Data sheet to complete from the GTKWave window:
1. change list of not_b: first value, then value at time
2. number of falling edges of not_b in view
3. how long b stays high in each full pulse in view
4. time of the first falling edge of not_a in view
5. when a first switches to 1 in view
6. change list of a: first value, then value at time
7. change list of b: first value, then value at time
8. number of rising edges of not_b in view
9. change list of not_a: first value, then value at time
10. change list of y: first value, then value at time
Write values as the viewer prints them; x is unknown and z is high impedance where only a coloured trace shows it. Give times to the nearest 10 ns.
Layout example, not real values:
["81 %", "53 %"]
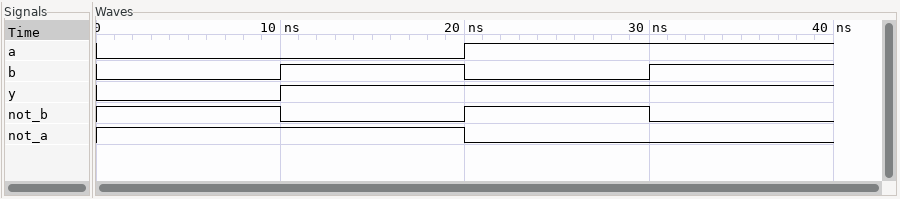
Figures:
["1, 0 at 10 ns, 1 at 20 ns, 0 at 30 ns", "2", "10 ns", "20 ns", "20 ns", "0, 1 at 20 ns", "0, 1 at 10 ns, 0 at 20 ns, 1 at 30 ns", "1", "1, 0 at 20 ns", "0, 1 at 10 ns"]
